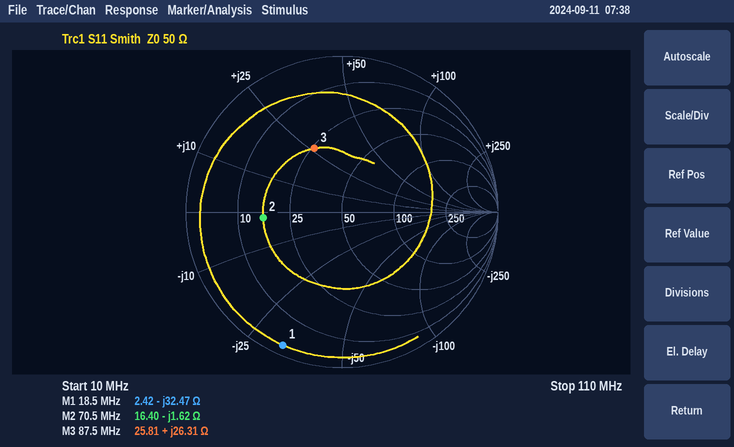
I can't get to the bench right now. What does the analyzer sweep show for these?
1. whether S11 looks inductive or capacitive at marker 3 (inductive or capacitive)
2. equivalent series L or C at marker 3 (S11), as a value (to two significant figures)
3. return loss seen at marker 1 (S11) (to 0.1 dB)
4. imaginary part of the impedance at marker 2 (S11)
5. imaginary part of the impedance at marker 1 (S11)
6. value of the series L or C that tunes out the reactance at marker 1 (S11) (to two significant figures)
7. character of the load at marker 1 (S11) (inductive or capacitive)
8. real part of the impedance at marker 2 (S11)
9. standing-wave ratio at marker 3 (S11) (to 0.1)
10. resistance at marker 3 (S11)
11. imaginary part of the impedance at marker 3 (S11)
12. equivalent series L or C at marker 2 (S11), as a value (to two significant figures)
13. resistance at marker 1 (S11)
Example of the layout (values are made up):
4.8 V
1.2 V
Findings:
inductive
48 nH
0.6 dB
-1.62 Ω
-32.47 Ω
280 nH
capacitive
16.40 Ω
2.6
25.81 Ω
+26.31 Ω
1.4 nF
2.42 Ω
